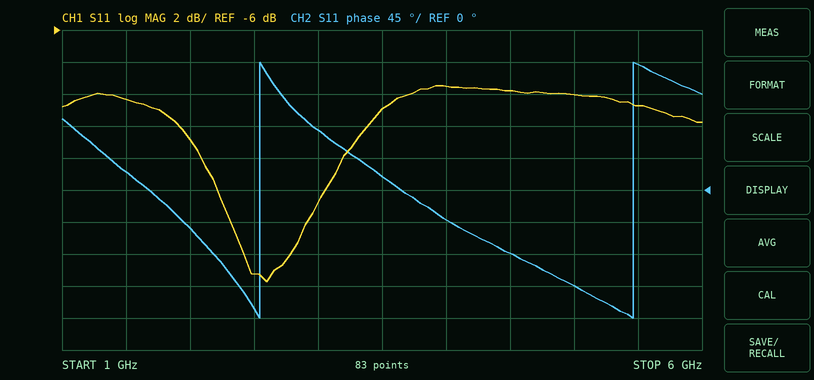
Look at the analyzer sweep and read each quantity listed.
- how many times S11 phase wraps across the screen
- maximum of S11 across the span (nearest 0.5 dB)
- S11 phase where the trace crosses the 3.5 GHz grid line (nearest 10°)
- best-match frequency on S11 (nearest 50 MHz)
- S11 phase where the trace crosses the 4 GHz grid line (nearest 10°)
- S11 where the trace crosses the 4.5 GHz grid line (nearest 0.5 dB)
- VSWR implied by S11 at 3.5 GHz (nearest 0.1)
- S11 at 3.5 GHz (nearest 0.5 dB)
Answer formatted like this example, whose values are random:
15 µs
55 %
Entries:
2
-9.5 dB
20°
2.60 GHz
-40°
-10.0 dB
1.8
-11.0 dB
